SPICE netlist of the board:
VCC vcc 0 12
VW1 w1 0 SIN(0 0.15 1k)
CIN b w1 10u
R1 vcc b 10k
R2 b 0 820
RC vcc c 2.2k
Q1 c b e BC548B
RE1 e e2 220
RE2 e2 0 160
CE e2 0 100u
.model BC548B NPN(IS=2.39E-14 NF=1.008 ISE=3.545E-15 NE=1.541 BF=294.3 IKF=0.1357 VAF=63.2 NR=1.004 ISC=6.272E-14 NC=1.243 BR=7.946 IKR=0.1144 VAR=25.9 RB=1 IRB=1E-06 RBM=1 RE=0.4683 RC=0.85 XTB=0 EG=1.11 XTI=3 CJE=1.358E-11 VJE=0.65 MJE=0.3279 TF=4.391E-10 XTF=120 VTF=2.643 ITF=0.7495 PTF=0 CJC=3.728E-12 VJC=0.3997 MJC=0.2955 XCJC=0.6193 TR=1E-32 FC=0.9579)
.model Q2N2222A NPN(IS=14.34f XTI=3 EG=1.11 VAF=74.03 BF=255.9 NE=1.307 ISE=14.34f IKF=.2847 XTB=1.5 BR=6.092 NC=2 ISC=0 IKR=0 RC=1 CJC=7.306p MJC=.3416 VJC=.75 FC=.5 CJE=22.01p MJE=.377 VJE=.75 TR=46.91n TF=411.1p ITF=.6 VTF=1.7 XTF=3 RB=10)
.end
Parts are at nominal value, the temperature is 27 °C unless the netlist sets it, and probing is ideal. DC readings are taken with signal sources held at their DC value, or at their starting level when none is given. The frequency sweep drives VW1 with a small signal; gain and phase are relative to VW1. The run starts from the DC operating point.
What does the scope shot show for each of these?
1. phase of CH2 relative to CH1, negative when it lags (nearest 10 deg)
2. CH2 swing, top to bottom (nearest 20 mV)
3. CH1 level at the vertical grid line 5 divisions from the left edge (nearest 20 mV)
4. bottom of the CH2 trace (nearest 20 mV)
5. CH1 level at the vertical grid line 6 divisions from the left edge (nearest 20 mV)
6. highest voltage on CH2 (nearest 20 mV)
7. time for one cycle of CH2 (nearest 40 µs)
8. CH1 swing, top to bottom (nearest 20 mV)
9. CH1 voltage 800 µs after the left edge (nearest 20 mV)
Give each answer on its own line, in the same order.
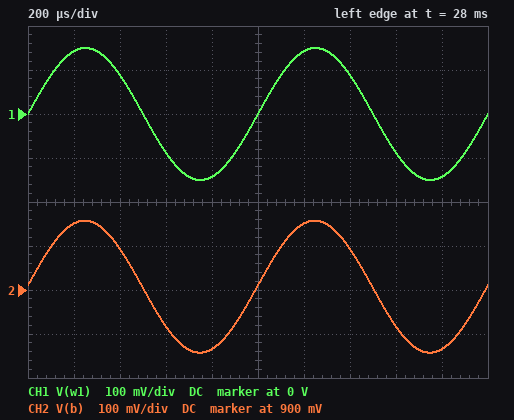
0 deg
300 mV
0 V
760 mV
140 mV
1.06 V
1.00 ms
300 mV
-140 mV
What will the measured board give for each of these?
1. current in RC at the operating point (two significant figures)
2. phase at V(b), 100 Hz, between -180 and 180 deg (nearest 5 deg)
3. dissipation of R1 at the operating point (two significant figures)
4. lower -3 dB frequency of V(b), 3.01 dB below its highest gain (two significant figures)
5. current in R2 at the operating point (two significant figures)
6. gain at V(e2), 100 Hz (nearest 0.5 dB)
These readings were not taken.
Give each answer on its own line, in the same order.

740 µA
10 deg
12 mW
21 Hz
1.1 mA
-24.5 dB
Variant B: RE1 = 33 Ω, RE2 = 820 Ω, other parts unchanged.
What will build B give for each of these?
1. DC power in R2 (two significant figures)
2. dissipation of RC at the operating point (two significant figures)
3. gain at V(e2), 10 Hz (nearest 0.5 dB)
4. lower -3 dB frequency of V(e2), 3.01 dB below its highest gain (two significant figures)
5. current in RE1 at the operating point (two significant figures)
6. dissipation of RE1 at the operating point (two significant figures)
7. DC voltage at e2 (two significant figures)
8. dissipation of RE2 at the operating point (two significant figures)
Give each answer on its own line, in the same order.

1.0 mW
270 µW
-10.0 dB
7.7 Hz
350 µA
4.1 µW
290 mV
100 µW
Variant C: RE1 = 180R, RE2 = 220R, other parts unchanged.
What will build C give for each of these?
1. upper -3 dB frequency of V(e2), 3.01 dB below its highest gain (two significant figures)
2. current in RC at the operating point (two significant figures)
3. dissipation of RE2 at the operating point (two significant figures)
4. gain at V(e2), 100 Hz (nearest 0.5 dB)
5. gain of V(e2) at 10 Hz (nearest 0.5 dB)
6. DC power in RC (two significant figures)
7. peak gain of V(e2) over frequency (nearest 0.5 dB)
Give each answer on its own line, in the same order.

43 Hz
700 µA
110 µW
-23.0 dB
-15.0 dB
1.1 mW
-14.0 dB
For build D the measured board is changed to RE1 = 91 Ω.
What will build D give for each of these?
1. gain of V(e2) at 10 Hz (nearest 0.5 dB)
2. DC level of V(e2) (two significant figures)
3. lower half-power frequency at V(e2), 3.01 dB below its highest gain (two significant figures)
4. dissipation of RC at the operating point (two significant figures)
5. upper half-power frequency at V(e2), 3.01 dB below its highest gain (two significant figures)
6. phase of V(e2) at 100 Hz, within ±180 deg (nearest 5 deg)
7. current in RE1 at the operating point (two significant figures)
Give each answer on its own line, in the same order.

-13.0 dB
170 mV
9.2 Hz
2.5 mW
54 Hz
-65 deg
1.1 mA
